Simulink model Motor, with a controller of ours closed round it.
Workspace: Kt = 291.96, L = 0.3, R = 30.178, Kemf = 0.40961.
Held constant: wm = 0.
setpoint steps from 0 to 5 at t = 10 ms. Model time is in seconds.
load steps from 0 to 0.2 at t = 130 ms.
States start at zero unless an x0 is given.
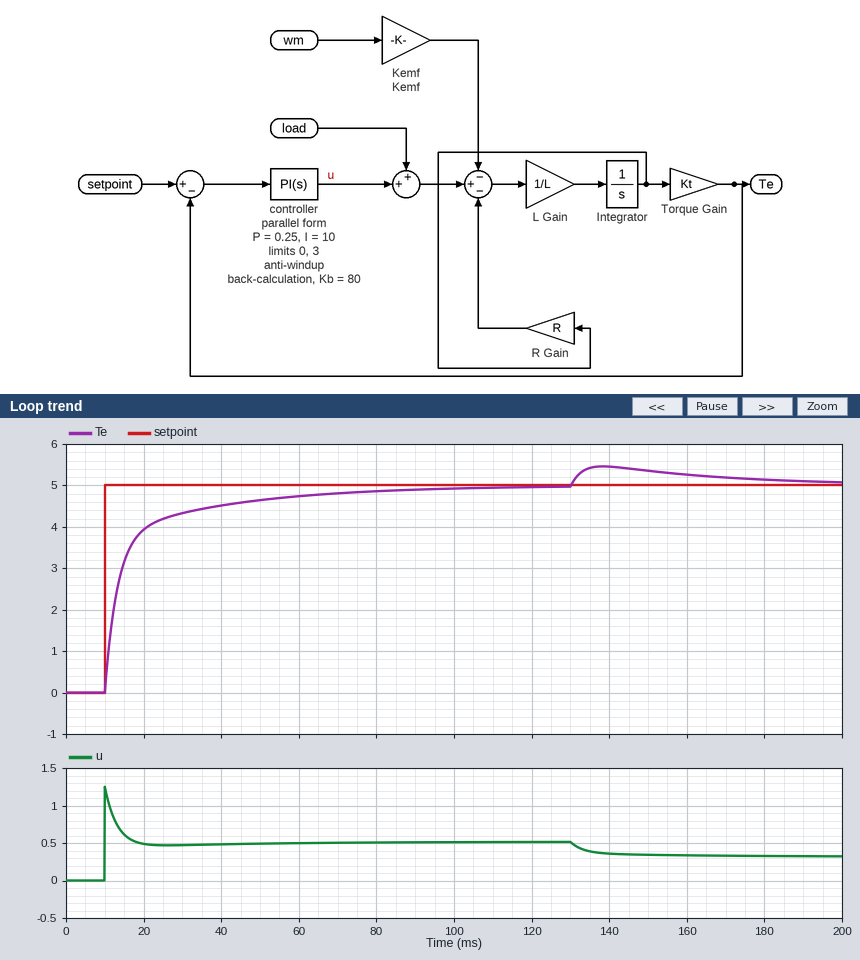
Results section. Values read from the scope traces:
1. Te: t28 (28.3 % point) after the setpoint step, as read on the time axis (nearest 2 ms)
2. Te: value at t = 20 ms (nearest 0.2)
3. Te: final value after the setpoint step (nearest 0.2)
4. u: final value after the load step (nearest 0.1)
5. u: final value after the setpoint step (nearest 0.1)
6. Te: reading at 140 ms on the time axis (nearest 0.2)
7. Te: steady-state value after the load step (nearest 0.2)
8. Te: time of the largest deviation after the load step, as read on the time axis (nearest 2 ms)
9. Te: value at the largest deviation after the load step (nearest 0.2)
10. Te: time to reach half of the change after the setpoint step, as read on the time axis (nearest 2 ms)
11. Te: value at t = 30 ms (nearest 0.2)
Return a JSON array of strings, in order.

["12 ms", "4.0", "5.0", "0.3", "0.5", "5.4", "5.0", "138 ms", "5.4", "14 ms", "4.4"]
